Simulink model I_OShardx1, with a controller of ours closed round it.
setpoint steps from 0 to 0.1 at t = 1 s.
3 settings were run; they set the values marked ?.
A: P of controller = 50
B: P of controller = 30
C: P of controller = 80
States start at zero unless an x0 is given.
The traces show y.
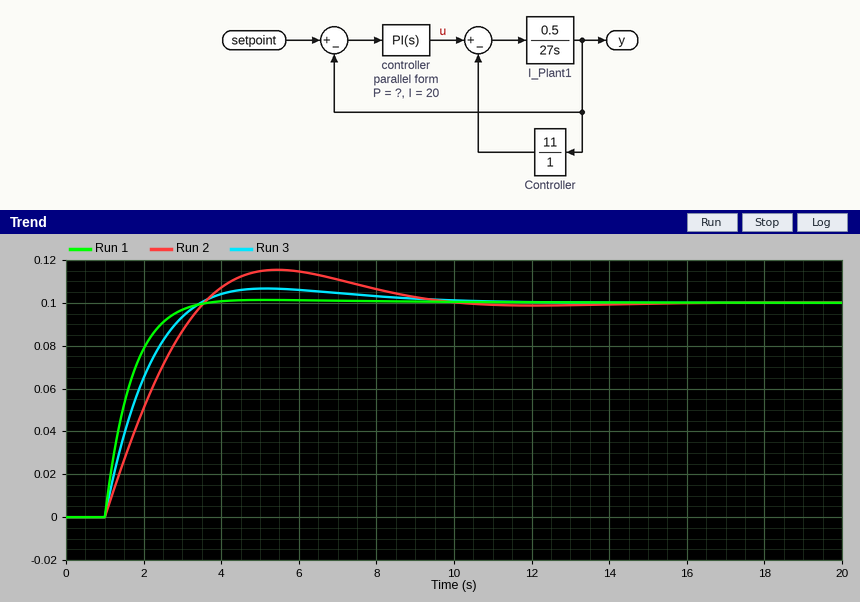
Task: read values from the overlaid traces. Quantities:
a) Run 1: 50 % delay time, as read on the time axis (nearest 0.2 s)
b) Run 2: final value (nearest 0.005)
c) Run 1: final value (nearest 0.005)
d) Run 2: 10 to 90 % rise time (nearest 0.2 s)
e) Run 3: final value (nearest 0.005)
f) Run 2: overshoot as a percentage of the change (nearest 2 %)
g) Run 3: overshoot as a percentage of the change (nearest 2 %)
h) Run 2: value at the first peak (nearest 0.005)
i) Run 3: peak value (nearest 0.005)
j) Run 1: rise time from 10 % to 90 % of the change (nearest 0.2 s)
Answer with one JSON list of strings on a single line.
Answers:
["1.4 s", "0.100", "0.100", "2.0 s", "0.100", "16 %", "6 %", "0.115", "0.105", "1.4 s"]
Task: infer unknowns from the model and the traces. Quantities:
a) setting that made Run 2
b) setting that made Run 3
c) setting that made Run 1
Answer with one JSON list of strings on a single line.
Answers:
["B", "A", "C"]
